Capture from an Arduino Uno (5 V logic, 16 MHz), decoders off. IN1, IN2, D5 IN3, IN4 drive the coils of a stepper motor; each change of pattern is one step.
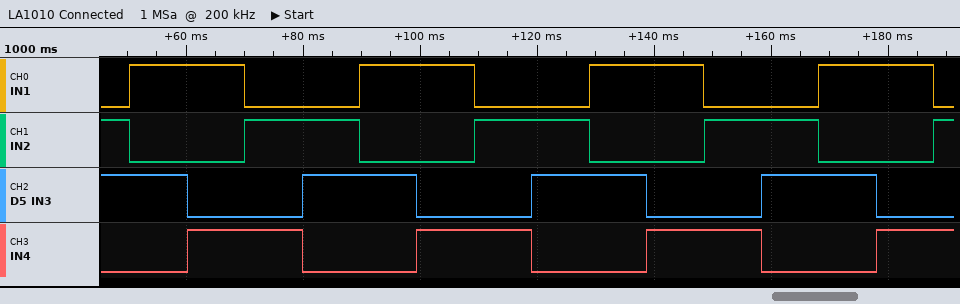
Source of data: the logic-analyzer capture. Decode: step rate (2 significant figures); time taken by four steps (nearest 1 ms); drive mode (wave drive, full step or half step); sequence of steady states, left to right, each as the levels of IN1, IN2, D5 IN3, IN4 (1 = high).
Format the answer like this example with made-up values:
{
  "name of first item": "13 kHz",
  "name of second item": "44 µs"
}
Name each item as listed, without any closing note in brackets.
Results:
{
  "step rate": "100 steps/s",
  "time taken by four steps": "39 ms",
  "drive mode": "full step",
  "sequence of steady states, left to right, each as the levels of IN1, IN2, D5 IN3, IN4": "0110 1010 1001 0101 0110 1010 1001 0101 0110 1010 1001 0101 0110 1010 1001 0101"
}
